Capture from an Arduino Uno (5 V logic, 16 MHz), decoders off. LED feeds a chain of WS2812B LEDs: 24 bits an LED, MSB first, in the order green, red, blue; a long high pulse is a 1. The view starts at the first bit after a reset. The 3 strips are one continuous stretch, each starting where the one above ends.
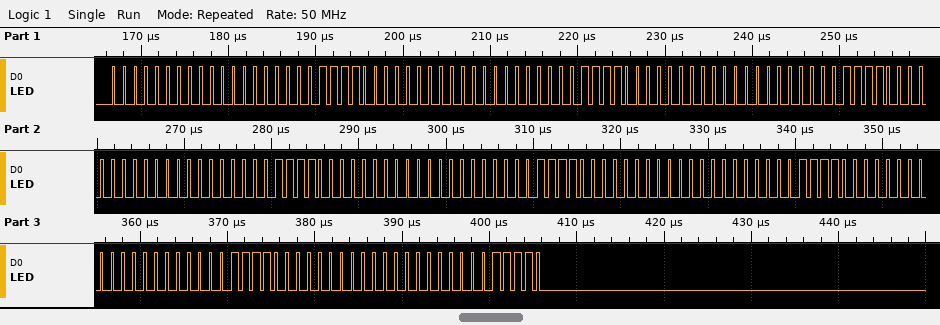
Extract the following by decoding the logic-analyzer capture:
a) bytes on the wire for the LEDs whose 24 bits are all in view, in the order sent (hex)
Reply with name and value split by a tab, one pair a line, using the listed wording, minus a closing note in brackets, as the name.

bytes on the wire for the LEDs whose 24 bits are all in view, in the order sent	00 00 1E 00 00 1E 00 00 1E 00 00 1E 00 00 1E 00 00 1E 00 00 1E 00 00 1E
